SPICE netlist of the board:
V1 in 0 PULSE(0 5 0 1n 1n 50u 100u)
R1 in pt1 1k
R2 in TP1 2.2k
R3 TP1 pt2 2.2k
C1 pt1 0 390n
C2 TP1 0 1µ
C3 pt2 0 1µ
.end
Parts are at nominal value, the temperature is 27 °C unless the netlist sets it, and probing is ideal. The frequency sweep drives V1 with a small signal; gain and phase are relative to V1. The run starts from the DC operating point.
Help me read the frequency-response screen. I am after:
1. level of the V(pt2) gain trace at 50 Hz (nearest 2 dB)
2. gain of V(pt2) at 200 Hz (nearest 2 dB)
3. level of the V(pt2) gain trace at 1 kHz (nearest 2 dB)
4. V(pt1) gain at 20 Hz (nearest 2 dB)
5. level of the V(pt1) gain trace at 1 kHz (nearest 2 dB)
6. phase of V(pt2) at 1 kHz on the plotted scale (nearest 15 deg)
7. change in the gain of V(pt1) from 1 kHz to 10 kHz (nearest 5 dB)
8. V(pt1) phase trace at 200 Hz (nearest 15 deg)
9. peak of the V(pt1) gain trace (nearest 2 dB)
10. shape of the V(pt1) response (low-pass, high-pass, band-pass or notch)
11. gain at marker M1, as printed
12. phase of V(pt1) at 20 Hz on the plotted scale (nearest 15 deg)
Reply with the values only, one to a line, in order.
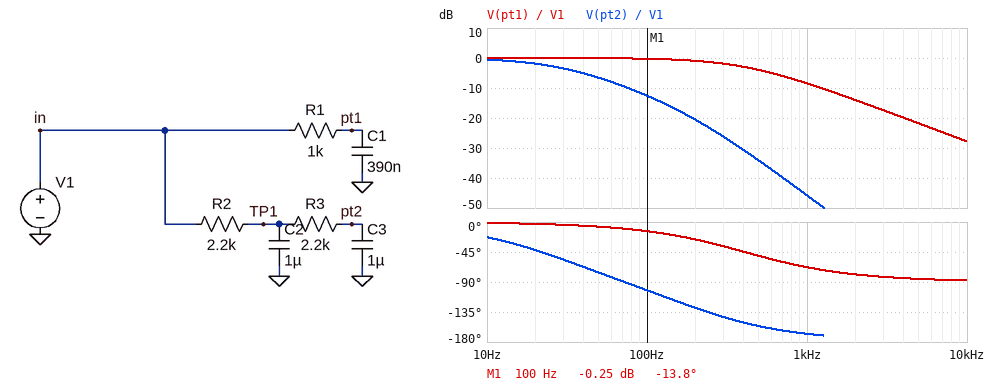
-6 dB
-20 dB
-46 dB
0 dB
-8 dB
-165 deg
-20 dB
-30 deg
0 dB
low-pass
-0.25 dB
0 deg
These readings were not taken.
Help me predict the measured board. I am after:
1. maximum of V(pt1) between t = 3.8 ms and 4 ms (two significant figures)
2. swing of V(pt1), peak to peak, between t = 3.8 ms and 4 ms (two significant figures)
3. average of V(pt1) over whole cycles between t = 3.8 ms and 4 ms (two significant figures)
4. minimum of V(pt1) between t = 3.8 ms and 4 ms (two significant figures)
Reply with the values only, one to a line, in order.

2.7 V
320 mV
2.5 V
2.3 V
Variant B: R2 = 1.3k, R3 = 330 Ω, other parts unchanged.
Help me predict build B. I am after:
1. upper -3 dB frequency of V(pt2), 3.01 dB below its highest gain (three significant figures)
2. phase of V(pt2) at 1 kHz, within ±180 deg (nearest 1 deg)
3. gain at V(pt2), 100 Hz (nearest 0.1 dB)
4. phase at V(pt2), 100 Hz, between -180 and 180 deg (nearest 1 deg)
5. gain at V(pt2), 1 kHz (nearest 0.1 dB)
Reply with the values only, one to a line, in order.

57.2 Hz
-131 deg
-6.1 dB
-66 deg
-27.7 dB
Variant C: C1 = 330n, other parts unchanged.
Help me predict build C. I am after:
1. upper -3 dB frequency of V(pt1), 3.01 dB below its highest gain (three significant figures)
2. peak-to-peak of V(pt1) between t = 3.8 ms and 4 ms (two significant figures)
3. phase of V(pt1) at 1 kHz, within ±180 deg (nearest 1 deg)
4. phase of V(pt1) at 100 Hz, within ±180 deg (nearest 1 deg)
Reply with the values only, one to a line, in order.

482 Hz
380 mV
-64 deg
-12 deg
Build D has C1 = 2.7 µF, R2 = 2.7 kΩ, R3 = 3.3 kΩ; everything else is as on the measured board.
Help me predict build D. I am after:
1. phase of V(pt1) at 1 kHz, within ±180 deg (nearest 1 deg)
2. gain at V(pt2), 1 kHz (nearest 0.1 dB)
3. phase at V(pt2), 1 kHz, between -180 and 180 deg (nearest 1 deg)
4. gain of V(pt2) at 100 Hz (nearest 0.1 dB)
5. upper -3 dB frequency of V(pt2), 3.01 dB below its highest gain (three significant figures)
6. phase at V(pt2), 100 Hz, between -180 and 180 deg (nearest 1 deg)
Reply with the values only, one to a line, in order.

-87 deg
-51.0 dB
-171 deg
-15.6 dB
20.7 Hz
-115 deg
